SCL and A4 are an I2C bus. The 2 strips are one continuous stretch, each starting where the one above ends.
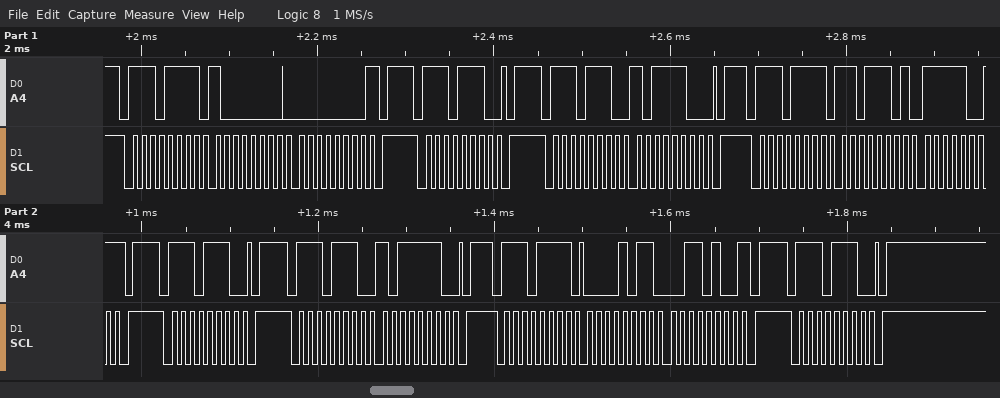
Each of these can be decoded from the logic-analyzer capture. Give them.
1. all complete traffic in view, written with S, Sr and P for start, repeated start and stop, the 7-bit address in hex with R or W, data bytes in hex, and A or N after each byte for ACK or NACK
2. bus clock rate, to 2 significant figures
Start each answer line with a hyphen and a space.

- S 77R A 80 A 00 N P S 77W A P S 77W A BC A P S 77R A DD A F9 N P S 77W A P S 77W A BE A P S 77R A 0B A 34 N P S 77W A P
- 100 kHz
